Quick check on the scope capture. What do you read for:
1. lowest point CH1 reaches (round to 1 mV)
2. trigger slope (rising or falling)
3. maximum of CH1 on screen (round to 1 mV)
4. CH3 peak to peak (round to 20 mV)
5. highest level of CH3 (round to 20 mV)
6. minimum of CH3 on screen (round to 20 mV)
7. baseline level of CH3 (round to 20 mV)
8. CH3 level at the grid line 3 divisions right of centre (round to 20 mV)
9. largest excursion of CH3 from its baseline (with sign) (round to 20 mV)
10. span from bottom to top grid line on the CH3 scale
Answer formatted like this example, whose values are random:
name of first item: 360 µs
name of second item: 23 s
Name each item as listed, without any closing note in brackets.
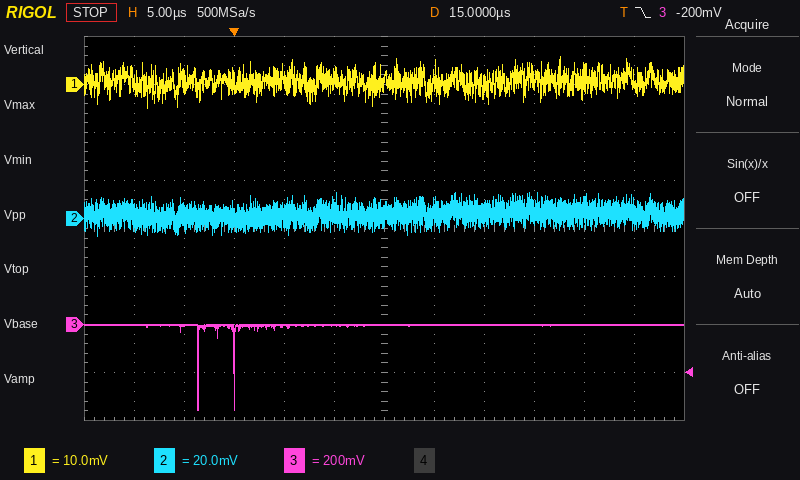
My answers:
lowest point CH1 reaches: -5 mV
trigger slope: falling
maximum of CH1 on screen: 6 mV
CH3 peak to peak: 360 mV
highest level of CH3: 0 mV
minimum of CH3 on screen: -360 mV
baseline level of CH3: 0 mV
CH3 level at the grid line 3 divisions right of centre: 0 mV
largest excursion of CH3 from its baseline (with sign): -360 mV
span from bottom to top grid line on the CH3 scale: 1.6 V
